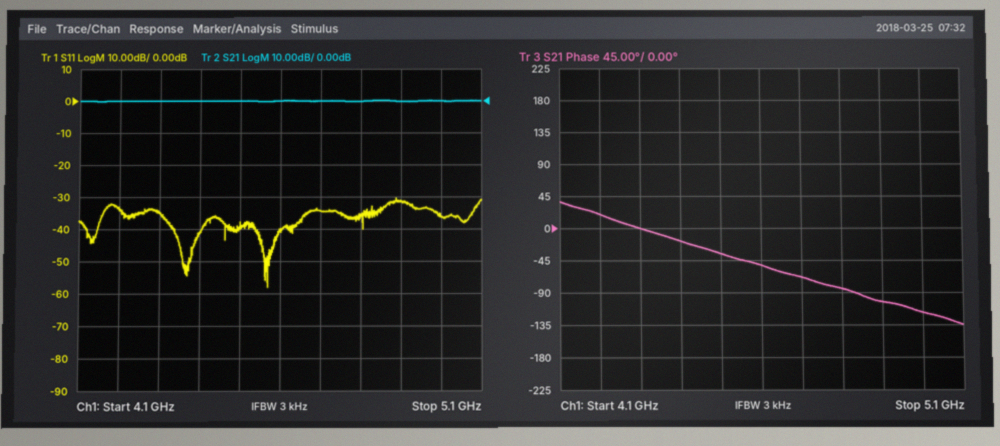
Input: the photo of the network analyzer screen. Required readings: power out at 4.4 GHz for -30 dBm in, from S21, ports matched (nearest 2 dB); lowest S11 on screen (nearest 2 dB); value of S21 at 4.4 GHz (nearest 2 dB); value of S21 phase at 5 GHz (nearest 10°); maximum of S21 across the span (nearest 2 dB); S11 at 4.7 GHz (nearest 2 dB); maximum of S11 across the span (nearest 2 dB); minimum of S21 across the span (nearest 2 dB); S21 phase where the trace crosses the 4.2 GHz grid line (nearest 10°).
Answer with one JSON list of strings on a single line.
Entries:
["-30 dBm", "-58 dB", "0 dB", "-120°", "0 dB", "-34 dB", "-30 dB", "0 dB", "20°"]
